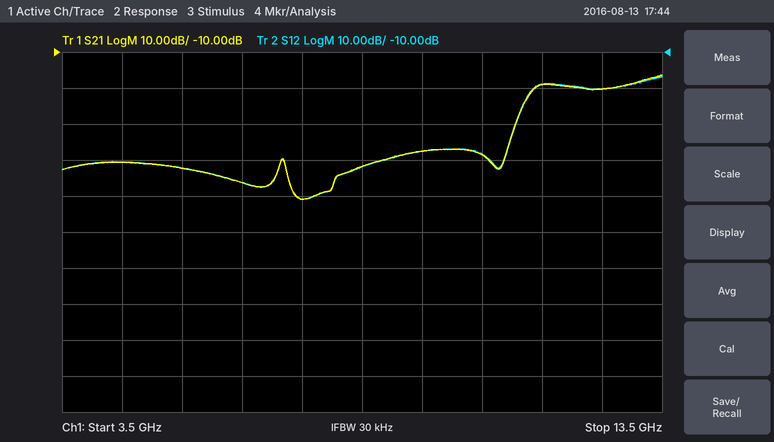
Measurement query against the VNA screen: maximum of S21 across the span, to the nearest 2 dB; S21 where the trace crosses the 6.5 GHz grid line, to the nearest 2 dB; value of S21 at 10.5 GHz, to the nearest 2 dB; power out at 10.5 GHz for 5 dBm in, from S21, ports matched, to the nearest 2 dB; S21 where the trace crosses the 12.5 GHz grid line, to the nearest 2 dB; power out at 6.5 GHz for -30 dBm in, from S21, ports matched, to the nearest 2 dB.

-16 dB
-46 dB
-38 dB
-34 dBm
-20 dB
-76 dBm
